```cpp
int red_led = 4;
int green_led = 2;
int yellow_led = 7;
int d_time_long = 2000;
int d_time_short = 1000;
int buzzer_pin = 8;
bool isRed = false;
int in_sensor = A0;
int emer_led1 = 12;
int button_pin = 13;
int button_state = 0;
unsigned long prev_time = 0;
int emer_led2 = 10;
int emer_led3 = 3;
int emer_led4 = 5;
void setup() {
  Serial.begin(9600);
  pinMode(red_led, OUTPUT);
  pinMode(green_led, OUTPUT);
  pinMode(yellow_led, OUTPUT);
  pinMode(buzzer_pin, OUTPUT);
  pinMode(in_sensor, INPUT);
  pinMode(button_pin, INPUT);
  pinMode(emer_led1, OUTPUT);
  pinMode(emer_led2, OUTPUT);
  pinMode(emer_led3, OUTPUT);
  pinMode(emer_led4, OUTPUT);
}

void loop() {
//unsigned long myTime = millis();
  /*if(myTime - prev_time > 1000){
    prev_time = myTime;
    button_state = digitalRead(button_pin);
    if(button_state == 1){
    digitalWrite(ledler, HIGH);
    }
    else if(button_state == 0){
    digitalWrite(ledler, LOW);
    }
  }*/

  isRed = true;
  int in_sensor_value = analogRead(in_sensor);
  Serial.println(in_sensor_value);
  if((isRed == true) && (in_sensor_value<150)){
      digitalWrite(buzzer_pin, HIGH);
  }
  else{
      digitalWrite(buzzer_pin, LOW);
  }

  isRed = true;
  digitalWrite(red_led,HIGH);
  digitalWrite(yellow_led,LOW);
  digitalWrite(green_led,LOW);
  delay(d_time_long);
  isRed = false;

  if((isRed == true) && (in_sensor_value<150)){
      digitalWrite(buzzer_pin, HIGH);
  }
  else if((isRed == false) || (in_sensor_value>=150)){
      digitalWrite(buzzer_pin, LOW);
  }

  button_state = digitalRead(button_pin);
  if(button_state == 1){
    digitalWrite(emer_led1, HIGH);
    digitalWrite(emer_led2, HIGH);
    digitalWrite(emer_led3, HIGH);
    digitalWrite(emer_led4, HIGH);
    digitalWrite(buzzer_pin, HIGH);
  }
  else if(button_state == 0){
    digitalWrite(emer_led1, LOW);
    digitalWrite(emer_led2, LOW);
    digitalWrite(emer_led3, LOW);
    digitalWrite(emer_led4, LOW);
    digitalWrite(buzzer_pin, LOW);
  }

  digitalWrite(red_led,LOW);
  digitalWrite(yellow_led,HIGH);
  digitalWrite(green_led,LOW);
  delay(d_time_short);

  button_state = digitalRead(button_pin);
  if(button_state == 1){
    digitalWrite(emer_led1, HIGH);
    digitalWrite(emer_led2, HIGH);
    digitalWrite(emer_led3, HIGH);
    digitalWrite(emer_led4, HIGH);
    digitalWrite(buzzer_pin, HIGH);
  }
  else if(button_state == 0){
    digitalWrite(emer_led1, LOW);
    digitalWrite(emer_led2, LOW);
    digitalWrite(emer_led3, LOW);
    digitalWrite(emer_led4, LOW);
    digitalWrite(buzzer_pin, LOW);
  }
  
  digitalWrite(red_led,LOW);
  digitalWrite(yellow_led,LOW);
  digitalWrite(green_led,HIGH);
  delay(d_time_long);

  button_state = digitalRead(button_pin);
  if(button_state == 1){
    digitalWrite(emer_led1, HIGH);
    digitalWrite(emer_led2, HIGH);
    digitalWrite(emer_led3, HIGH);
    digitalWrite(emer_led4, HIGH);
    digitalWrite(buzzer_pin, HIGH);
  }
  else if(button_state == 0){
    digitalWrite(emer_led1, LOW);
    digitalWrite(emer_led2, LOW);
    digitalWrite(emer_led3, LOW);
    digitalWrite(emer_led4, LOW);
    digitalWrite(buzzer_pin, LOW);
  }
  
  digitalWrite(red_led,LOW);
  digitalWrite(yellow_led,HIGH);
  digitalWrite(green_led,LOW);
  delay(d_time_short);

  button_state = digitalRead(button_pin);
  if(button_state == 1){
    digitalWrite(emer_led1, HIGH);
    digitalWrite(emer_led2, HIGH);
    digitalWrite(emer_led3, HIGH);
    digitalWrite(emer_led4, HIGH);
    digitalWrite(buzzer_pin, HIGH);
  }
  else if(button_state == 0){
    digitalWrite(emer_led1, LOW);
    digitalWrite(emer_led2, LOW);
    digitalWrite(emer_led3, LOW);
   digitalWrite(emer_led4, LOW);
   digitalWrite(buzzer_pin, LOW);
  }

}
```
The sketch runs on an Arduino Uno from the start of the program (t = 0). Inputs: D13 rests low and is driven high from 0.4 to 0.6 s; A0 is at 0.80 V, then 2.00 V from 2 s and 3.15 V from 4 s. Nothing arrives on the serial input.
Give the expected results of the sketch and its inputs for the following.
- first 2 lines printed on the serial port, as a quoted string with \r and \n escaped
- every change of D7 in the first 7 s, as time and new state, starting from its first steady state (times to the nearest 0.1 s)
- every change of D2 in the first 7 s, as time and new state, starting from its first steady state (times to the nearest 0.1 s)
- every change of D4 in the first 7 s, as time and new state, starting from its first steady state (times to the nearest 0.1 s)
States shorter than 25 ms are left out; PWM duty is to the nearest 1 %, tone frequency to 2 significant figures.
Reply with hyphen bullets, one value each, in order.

- "163\r\n645\r\n"
- 0 s low; 2 s high; 3 s low; 5 s high; 6 s low
- 0 s low; 3 s high; 5 s low
- 0 s high; 2 s low; 6 s high
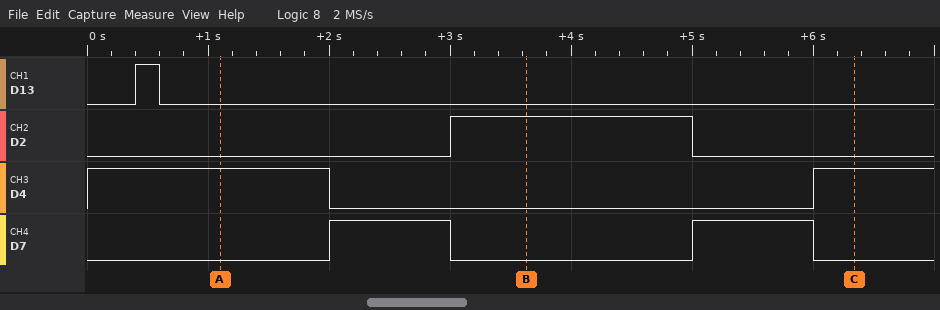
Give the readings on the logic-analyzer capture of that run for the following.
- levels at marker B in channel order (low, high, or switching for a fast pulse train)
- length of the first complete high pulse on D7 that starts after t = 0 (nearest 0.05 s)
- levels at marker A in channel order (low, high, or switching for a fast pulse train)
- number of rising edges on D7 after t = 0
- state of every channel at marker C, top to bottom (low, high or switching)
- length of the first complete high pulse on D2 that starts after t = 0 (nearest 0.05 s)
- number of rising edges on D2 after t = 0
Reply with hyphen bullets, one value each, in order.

- D13 low, D2 high, D4 low, D7 low
- 1.00 s
- D13 low, D2 low, D4 high, D7 low
- 2
- D13 low, D2 low, D4 high, D7 low
- 2.00 s
- 1
